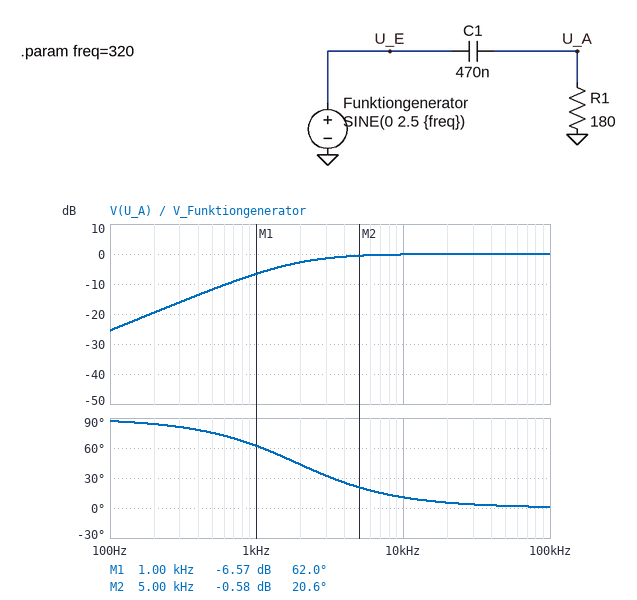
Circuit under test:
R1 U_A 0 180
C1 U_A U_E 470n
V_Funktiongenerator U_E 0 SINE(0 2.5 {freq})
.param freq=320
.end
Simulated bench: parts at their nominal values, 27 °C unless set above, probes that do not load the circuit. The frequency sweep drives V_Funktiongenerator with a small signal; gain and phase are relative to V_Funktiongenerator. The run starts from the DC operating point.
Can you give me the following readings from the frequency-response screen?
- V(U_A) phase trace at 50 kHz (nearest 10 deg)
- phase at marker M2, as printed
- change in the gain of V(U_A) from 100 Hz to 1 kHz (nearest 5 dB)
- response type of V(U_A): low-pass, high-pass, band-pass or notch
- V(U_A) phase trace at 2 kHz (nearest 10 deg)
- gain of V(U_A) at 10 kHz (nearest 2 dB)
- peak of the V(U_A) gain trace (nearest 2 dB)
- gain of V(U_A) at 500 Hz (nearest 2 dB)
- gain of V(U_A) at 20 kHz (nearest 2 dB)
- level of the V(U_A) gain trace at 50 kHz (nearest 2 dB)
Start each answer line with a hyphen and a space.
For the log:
- 0 deg
- 20.6 deg
- 20 dB
- high-pass
- 40 deg
- 0 dB
- 0 dB
- -12 dB
- 0 dB
- 0 dB
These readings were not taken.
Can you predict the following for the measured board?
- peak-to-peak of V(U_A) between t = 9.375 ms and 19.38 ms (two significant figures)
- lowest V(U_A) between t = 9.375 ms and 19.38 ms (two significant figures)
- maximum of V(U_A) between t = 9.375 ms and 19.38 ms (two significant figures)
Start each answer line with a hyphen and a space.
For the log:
- 840 mV
- -420 mV
- 420 mV
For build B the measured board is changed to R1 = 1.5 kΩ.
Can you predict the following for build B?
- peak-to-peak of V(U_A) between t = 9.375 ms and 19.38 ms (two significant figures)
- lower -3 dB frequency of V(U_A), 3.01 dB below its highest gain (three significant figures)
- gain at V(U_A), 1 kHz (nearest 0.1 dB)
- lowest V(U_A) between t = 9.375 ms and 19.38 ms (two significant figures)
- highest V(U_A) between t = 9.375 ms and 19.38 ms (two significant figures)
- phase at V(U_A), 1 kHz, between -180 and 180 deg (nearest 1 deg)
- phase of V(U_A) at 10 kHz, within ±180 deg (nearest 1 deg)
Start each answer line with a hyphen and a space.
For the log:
- 4.1 V
- 226 Hz
- -0.2 dB
- -2.0 V
- 2.0 V
- 13 deg
- 1 deg
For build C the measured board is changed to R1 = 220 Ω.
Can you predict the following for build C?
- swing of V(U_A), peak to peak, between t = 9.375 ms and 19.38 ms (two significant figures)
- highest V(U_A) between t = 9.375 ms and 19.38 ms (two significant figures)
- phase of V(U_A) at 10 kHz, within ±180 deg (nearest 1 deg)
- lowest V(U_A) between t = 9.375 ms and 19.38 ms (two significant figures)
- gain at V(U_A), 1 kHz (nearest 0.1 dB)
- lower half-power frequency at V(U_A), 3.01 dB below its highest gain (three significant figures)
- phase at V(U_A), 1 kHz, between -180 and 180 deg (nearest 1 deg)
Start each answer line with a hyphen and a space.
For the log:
- 1.0 V
- 510 mV
- 9 deg
- -510 mV
- -5.3 dB
- 1.54 kHz
- 57 deg
